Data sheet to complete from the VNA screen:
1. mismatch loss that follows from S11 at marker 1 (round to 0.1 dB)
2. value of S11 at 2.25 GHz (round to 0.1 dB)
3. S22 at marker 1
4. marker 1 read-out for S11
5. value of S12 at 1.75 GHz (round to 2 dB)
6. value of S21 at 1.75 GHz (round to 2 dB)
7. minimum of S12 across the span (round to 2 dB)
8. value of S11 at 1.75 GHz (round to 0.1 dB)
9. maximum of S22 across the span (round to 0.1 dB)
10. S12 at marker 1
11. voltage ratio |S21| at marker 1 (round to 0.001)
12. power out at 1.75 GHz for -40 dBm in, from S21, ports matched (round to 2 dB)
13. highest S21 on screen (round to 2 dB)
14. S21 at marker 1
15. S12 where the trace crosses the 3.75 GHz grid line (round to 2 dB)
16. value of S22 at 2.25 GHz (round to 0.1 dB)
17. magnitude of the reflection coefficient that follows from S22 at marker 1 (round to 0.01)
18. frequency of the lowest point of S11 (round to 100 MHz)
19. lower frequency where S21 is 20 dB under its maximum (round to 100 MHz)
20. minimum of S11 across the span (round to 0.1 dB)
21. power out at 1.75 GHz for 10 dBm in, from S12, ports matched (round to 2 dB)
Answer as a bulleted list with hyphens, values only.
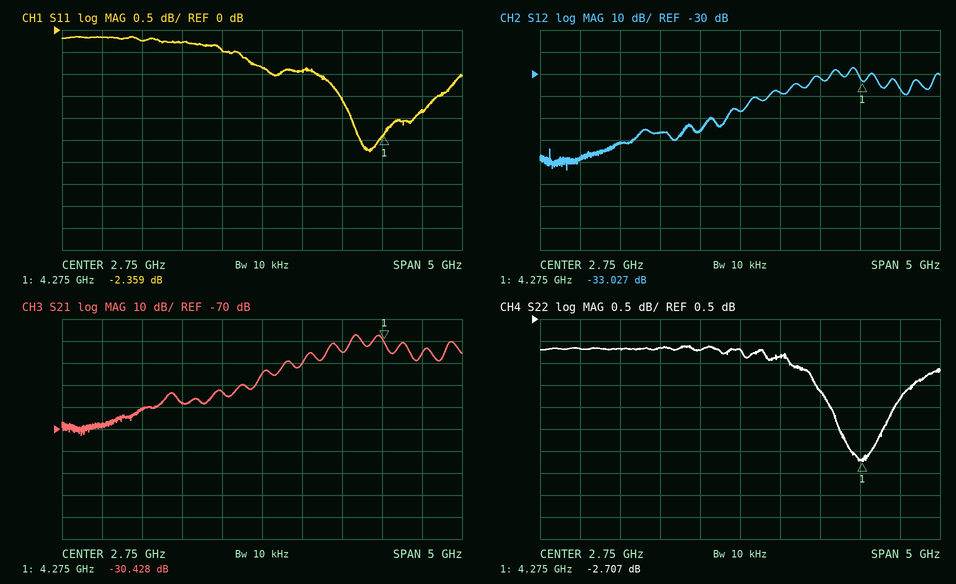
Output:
- 3.8 dB
- -0.5 dB
- -2.707 dB
- -2.359 dB
- -56 dB
- -58 dB
- -74 dB
- -0.3 dB
- -0.1 dB
- -33.027 dB
- 0.030
- -98 dBm
- -28 dB
- -30.428 dB
- -32 dB
- -0.2 dB
- 0.73
- 4.1 GHz
- 2.7 GHz
- -2.8 dB
- -46 dBm
